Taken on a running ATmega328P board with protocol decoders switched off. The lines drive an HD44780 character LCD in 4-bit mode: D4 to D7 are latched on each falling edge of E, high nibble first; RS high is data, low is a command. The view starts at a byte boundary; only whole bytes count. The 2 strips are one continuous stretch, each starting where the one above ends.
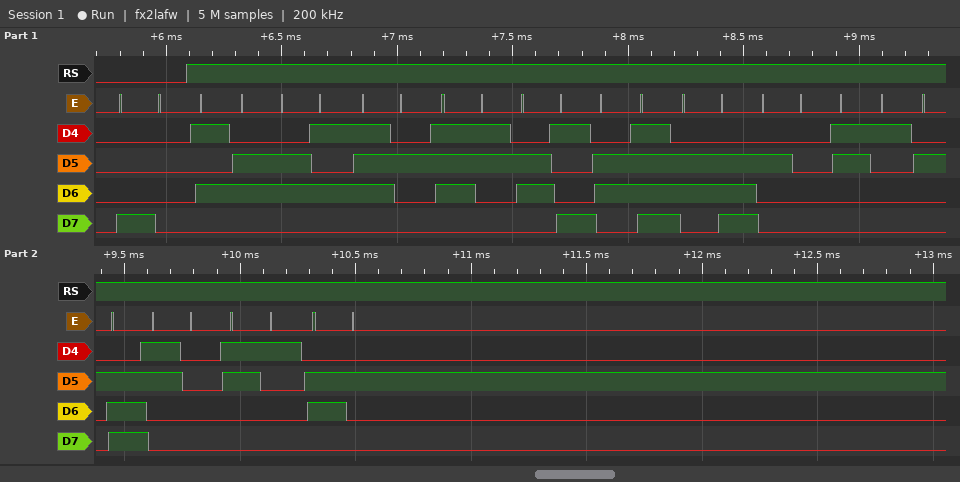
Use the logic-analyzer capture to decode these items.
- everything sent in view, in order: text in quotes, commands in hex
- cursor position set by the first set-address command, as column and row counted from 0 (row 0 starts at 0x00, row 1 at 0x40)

0x80 "Version 1.01b"
column 0, row 0
